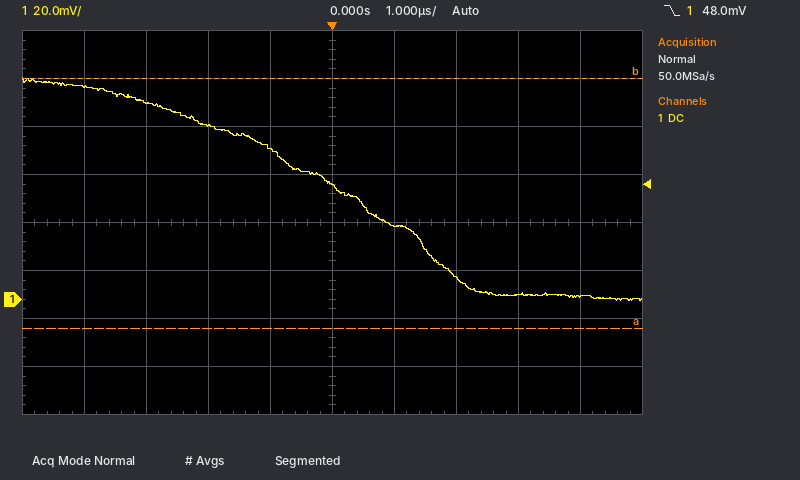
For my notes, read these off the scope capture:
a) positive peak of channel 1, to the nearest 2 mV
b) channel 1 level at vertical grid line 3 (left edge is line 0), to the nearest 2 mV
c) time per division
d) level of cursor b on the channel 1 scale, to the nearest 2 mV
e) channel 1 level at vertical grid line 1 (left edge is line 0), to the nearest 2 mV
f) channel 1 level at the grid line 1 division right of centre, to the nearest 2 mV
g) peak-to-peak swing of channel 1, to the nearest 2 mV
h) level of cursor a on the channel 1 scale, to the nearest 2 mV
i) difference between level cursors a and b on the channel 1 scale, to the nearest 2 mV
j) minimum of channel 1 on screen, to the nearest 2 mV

92 mV
72 mV
1 µs
92 mV
88 mV
30 mV
92 mV
-12 mV
104 mV
0 mV
